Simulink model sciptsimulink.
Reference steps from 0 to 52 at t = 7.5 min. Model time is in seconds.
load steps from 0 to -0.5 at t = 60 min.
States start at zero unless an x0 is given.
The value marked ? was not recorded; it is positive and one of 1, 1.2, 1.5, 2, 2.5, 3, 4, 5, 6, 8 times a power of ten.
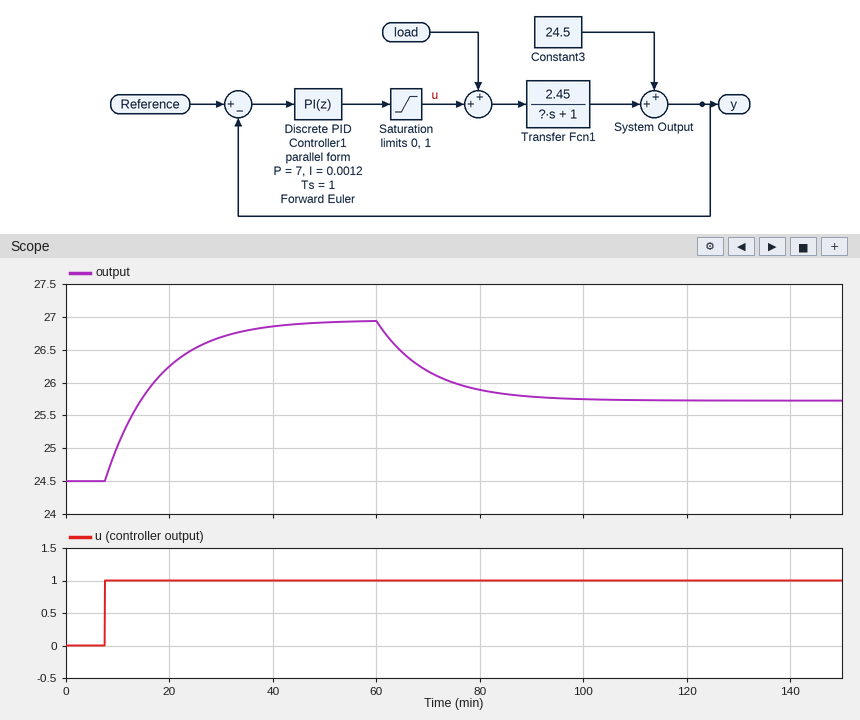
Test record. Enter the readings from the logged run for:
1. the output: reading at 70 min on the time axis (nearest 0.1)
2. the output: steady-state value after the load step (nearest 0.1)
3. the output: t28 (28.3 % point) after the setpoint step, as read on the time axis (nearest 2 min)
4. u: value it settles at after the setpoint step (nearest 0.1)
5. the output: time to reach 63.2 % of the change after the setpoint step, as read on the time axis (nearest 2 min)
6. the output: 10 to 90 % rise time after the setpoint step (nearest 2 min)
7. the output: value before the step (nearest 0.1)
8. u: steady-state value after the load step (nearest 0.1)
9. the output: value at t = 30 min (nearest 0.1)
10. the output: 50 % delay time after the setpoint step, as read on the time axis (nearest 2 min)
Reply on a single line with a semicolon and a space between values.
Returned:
26.2; 25.7; 10 min; 1.0; 18 min; 22 min; 24.5; 1.0; 26.7; 14 min
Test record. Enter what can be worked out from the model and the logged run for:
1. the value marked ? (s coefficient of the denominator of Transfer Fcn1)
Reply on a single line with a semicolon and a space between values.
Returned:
600
